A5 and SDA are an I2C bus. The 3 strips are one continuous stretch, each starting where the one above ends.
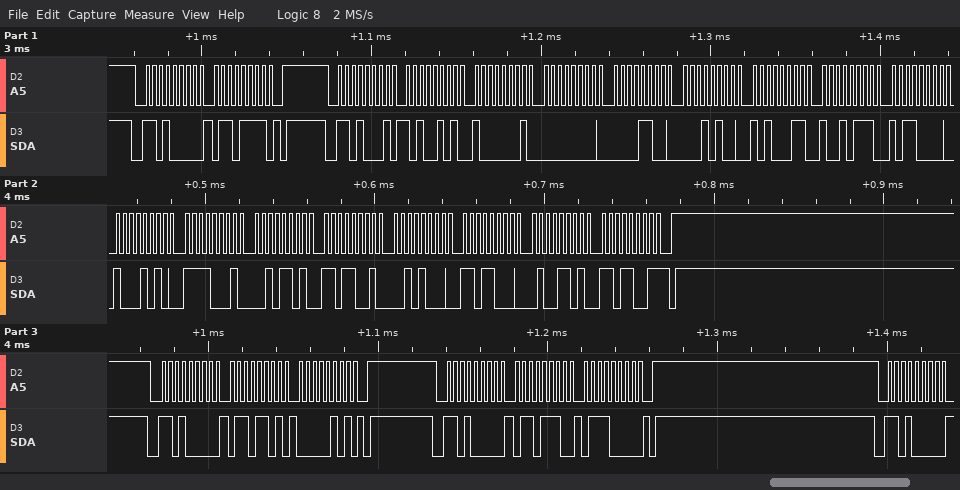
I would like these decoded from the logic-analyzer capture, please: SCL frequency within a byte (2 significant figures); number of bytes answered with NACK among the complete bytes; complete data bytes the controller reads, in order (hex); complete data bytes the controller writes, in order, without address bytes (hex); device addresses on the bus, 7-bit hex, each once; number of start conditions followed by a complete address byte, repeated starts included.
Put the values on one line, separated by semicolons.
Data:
250 kHz; 1; A5 81 00 0C 14 A3 97 B0 8A F1 2D D9 28 D8 4D D9; 6F 6D 05 6E 70; 0x68; 5
